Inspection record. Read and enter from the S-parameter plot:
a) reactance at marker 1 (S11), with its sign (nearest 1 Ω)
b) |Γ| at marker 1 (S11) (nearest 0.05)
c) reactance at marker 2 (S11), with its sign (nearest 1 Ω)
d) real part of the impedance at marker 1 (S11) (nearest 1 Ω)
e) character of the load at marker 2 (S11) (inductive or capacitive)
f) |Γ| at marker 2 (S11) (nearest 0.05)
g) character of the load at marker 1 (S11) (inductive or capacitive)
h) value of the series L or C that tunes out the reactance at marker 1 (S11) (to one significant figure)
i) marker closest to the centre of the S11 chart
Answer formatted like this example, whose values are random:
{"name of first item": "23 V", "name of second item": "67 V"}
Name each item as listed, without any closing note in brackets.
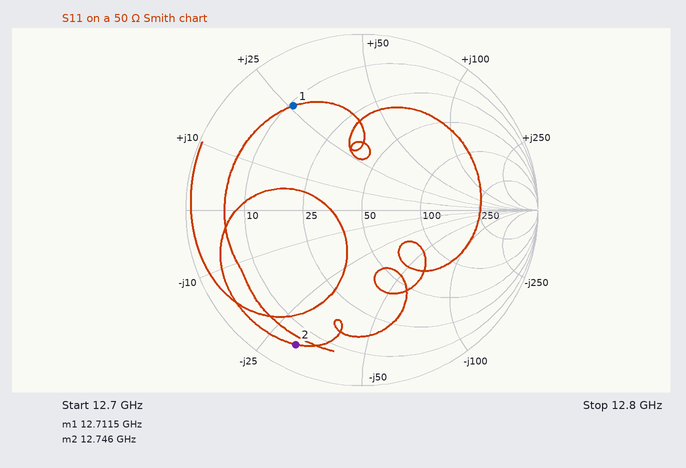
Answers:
{"reactance at marker 1 (S11), with its sign": "+26 Ω", "|Γ| at marker 1 (S11)": "0.70", "reactance at marker 2 (S11), with its sign": "-31 Ω", "real part of the impedance at marker 1 (S11)": "11 Ω", "character of the load at marker 2 (S11)": "capacitive", "|Γ| at marker 2 (S11)": "0.85", "character of the load at marker 1 (S11)": "inductive", "value of the series L or C that tunes out the reactance at marker 1 (S11)": "500 fF", "marker closest to the centre of the S11 chart": "marker 1"}
